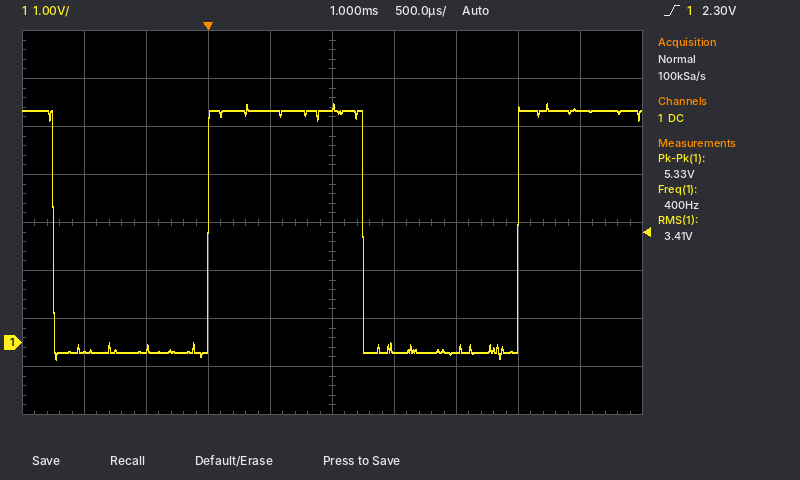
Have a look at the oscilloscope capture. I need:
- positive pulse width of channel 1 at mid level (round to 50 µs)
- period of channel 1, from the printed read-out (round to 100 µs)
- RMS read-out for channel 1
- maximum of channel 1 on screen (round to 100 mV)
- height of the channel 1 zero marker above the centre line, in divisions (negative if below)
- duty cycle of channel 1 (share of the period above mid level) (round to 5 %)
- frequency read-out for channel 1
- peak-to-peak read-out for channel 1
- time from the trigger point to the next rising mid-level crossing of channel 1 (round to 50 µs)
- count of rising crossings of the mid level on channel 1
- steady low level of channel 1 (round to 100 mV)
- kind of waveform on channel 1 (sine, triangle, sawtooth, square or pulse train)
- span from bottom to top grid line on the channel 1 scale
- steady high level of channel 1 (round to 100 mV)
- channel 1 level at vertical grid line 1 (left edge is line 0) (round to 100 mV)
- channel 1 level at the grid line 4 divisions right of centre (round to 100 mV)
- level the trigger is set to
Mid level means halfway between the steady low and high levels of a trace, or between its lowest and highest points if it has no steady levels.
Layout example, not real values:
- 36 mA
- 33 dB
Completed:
- 1.25 ms
- 2.5 ms
- 3.41 V
- 5.0 V
- -2.5 div
- 50 %
- 400 Hz
- 5.33 V
- 2.50 ms
- 2
- -200 mV
- square
- 8 V
- 4.8 V
- -200 mV
- 4.8 V
- 2.30 V
